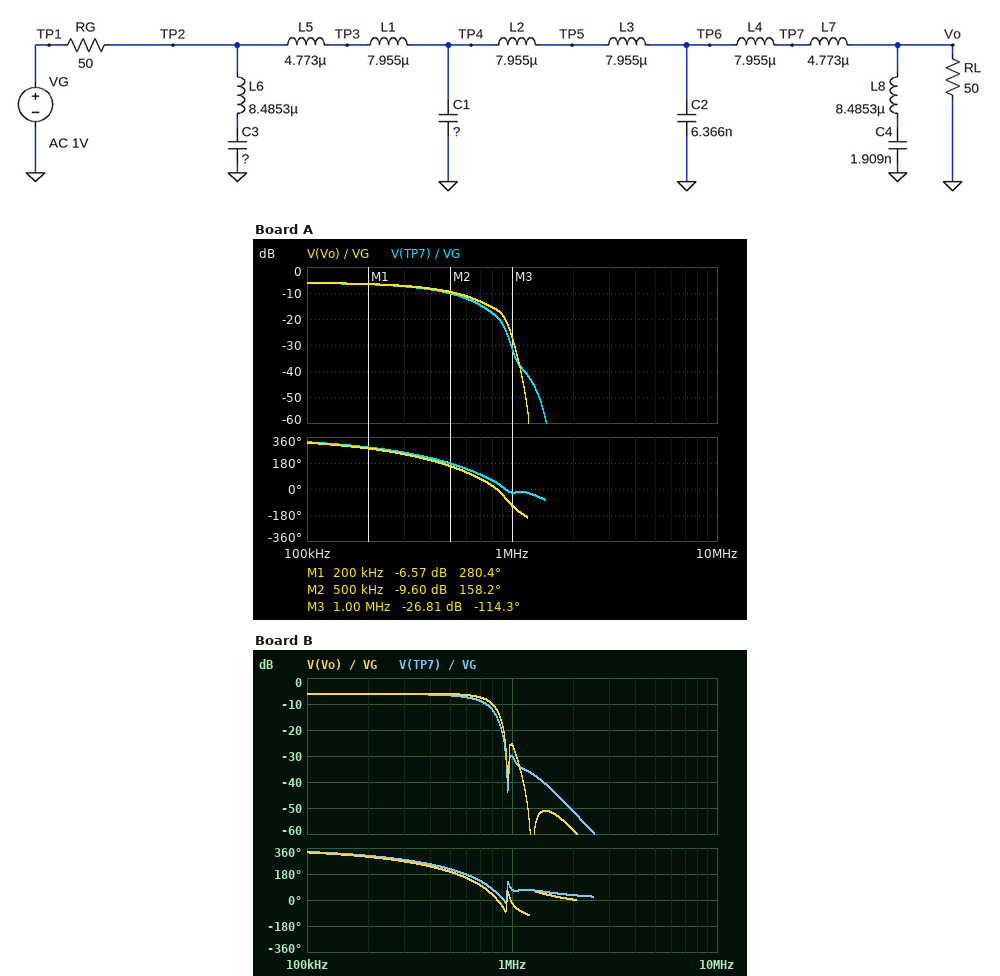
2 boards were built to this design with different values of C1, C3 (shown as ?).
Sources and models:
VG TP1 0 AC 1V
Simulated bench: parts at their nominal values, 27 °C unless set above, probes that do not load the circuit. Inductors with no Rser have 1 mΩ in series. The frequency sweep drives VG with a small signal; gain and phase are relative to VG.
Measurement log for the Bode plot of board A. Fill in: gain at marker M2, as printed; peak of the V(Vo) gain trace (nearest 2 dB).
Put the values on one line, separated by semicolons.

-9.60 dB; -6 dB
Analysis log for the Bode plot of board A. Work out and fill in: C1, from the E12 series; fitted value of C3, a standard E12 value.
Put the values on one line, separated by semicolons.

18 nF; 1.2 nF
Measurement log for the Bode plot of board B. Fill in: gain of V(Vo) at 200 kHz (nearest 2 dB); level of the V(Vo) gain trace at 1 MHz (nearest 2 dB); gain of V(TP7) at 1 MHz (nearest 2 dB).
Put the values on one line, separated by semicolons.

-6 dB; -26 dB; -30 dB
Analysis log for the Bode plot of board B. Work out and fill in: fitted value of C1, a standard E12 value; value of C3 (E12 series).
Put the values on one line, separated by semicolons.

5.6 nF; 3.3 nF
